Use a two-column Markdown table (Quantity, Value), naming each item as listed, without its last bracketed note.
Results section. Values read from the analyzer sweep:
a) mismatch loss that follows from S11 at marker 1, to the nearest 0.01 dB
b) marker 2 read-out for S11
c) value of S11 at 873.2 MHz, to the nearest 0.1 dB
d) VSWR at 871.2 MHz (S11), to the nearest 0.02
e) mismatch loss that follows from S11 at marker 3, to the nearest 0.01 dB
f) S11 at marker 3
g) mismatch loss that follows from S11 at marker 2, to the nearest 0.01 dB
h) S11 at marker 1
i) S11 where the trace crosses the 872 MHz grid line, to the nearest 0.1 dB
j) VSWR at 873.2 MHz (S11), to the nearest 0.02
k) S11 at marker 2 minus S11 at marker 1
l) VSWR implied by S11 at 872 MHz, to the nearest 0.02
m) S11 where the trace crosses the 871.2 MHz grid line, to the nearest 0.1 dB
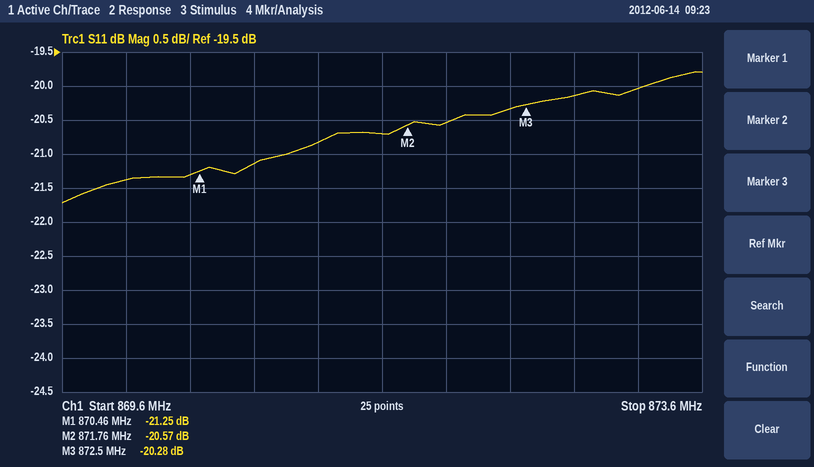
| Quantity | Value |
|---|---|
| mismatch loss that follows from S11 at marker 1, to the nearest 0.01 dB | 0.03 dB |
| marker 2 read-out for S11 | -20.57 dB |
| value of S11 at 873.2 MHz, to the nearest 0.1 dB | -20.0 dB |
| VSWR at 871.2 MHz (S11), to the nearest 0.02 | 1.20 |
| mismatch loss that follows from S11 at marker 3, to the nearest 0.01 dB | 0.04 dB |
| S11 at marker 3 | -20.28 dB |
| mismatch loss that follows from S11 at marker 2, to the nearest 0.01 dB | 0.04 dB |
| S11 at marker 1 | -21.25 dB |
| S11 where the trace crosses the 872 MHz grid line, to the nearest 0.1 dB | -20.5 dB |
| VSWR at 873.2 MHz (S11), to the nearest 0.02 | 1.22 |
| S11 at marker 2 minus S11 at marker 1 | 0.68 dB |
| VSWR implied by S11 at 872 MHz, to the nearest 0.02 | 1.20 |
| S11 where the trace crosses the 871.2 MHz grid line, to the nearest 0.1 dB | -20.8 dB |
